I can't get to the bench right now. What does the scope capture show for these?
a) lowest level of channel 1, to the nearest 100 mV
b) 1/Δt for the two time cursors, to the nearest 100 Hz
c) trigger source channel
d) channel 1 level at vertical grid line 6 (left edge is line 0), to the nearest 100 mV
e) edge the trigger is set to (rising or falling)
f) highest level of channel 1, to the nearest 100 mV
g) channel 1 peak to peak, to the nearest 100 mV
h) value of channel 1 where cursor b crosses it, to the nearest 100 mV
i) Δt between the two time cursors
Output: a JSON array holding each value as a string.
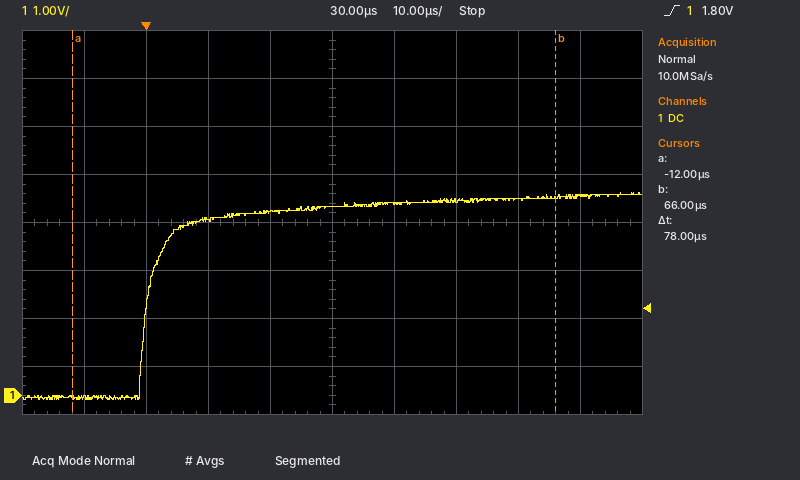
["-100 mV", "12.8 kHz", "channel 1", "4.0 V", "rising", "4.2 V", "4.3 V", "4.1 V", "78 µs"]
